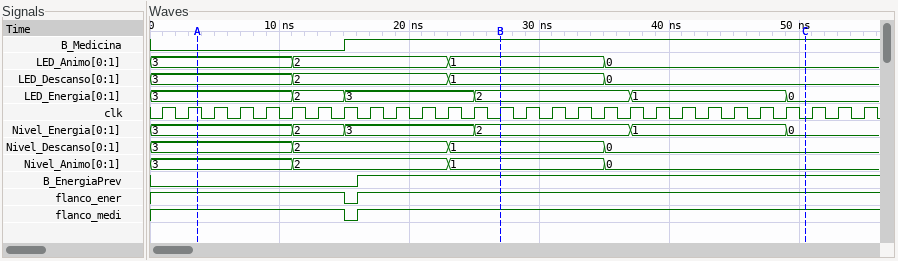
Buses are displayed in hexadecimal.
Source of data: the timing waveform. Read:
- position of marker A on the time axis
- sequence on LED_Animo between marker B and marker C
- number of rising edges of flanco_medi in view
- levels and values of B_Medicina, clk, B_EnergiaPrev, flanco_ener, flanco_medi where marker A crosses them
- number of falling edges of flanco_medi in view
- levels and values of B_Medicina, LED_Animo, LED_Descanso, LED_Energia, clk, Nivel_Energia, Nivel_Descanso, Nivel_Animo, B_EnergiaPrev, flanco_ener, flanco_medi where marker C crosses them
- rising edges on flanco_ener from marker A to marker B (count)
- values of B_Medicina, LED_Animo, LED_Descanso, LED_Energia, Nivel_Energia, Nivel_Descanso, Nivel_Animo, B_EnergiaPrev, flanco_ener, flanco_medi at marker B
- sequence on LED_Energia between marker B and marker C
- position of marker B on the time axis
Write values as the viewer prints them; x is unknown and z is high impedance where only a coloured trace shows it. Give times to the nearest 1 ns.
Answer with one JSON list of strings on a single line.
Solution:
["4 ns", "1, 0", "1", "B_Medicina=0, clk=1, B_EnergiaPrev=0, flanco_ener=1, flanco_medi=1", "1", "B_Medicina=1, LED_Animo=0, LED_Descanso=0, LED_Energia=0, clk=0, Nivel_Energia=0, Nivel_Descanso=0, Nivel_Animo=0, B_EnergiaPrev=1, flanco_ener=1, flanco_medi=1", "1", "B_Medicina=1, LED_Animo=1, LED_Descanso=1, LED_Energia=2, Nivel_Energia=2, Nivel_Descanso=1, Nivel_Animo=1, B_EnergiaPrev=1, flanco_ener=1, flanco_medi=1", "2, 1, 0", "27 ns"]
